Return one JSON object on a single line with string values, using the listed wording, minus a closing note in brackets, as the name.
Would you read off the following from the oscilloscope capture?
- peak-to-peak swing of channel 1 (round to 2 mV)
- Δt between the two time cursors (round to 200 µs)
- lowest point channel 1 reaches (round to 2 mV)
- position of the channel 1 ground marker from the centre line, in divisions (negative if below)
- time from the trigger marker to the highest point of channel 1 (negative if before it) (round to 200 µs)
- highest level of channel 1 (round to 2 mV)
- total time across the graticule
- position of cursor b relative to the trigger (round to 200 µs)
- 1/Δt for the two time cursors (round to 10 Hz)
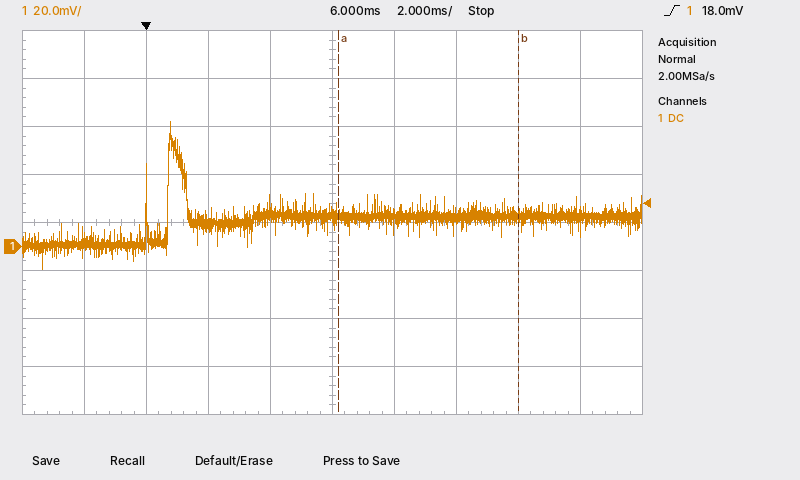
{"peak-to-peak swing of channel 1": "62 mV", "Δt between the two time cursors": "5.8 ms", "lowest point channel 1 reaches": "-10 mV", "position of the channel 1 ground marker from the centre line, in divisions": "-0.5 div", "time from the trigger marker to the highest point of channel 1 (negative if before it)": "+800 µs", "highest level of channel 1": "52 mV", "total time across the graticule": "20 ms", "position of cursor b relative to the trigger": "+12.0 ms", "1/Δt for the two time cursors": "170 Hz"}
